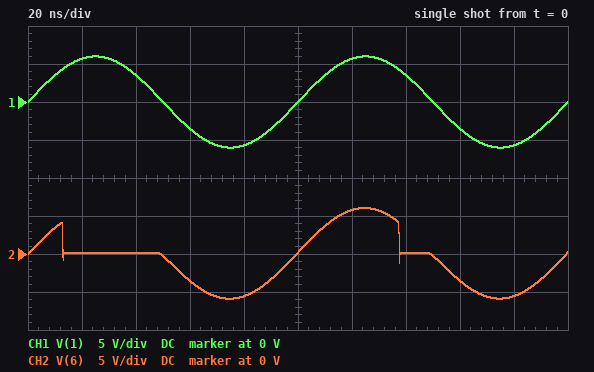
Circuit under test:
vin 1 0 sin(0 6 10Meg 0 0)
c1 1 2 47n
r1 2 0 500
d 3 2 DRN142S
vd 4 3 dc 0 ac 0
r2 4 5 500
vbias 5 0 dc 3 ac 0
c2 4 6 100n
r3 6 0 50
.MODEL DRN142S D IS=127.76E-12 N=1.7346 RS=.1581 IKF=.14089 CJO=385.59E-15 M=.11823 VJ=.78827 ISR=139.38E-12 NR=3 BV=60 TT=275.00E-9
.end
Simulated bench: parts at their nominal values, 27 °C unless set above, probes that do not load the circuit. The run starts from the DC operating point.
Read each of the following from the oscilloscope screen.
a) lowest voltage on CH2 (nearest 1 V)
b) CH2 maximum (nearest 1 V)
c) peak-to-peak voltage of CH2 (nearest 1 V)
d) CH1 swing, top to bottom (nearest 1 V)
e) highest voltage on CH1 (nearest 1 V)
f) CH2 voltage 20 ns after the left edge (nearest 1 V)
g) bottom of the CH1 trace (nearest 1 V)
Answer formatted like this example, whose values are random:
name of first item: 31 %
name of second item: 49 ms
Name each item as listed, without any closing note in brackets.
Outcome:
lowest voltage on CH2: -6 V
CH2 maximum: 6 V
peak-to-peak voltage of CH2: 12 V
CH1 swing, top to bottom: 12 V
highest voltage on CH1: 6 V
CH2 voltage 20 ns after the left edge: 0 V
bottom of the CH1 trace: -6 V
